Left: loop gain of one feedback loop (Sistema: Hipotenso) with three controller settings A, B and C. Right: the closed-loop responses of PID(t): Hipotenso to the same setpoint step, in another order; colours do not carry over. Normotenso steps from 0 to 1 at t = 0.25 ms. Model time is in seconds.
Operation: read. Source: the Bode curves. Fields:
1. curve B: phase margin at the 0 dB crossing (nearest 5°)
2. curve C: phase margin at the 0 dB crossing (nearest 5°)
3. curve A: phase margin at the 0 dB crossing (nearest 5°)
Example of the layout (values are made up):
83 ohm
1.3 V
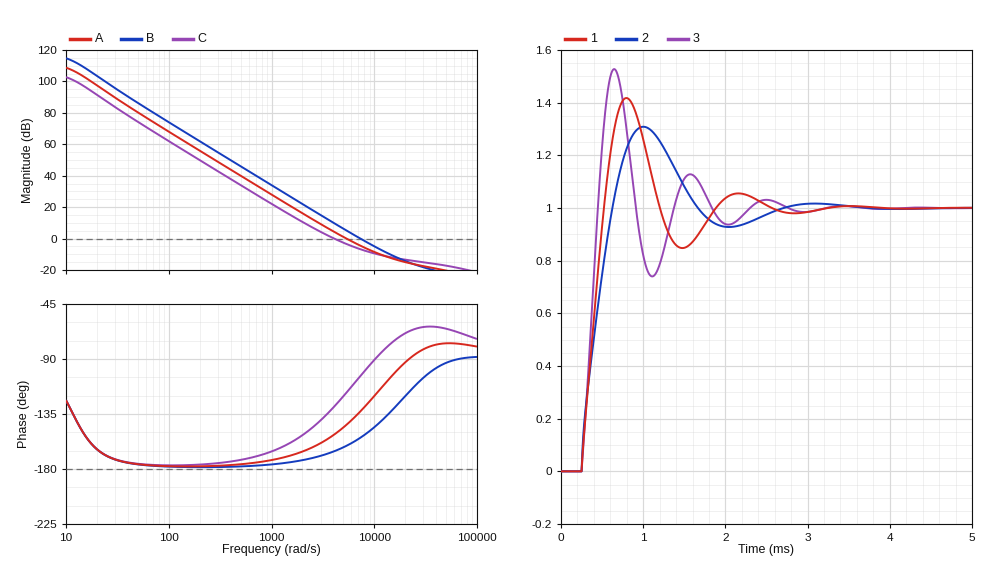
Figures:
25°
50°
35°
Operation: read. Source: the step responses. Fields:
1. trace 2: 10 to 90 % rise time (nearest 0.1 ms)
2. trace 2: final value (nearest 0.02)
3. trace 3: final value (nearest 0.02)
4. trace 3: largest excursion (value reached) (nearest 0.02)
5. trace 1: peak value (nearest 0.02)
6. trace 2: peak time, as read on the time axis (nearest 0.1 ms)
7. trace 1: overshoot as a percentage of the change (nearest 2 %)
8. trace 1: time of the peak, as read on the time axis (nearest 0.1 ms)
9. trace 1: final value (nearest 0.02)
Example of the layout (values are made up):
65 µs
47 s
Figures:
0.3 ms
1.00
1.00
1.52
1.42
1.0 ms
42 %
0.8 ms
1.00
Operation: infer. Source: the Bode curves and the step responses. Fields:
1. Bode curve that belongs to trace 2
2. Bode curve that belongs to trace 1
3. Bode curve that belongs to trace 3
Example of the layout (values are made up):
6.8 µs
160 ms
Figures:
C
A
B
